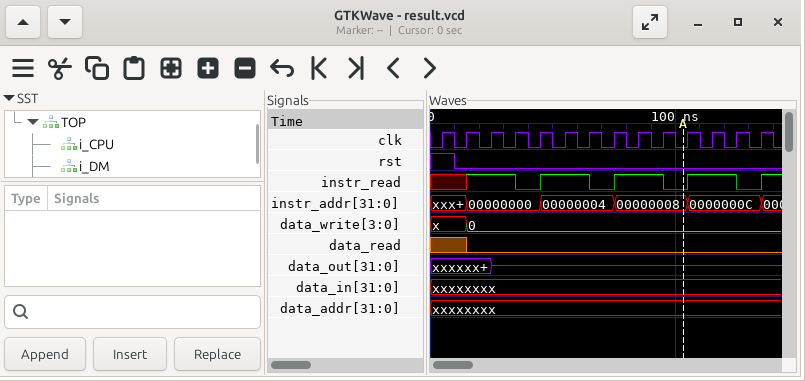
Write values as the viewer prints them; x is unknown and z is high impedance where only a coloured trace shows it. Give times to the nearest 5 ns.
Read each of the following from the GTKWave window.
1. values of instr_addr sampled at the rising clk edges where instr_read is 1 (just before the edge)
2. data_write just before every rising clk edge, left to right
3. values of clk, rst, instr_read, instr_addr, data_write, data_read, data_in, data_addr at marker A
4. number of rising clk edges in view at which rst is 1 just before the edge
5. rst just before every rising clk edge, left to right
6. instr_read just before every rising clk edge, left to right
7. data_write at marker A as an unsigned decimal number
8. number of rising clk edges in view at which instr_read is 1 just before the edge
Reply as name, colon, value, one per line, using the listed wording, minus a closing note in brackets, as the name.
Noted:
values of instr_addr sampled at the rising clk edges where instr_read is 1: 00000000, 00000000, 00000004, 00000004, 00000008, 00000008, 0000000C, 0000000C
data_write just before every rising clk edge, left to right: x, x, 0, 0, 0, 0, 0, 0, 0, 0, 0, 0, 0, 0
values of clk, rst, instr_read, instr_addr, data_write, data_read, data_in, data_addr at marker A: clk=0, rst=0, instr_read=0, instr_addr=00000008, data_write=0, data_read=0, data_in=xxxxxxxx, data_addr=xxxxxxxx
number of rising clk edges in view at which rst is 1 just before the edge: 1
rst just before every rising clk edge, left to right: 1 0 0 0 0 0 0 0 0 0 0 0 0 0
instr_read just before every rising clk edge, left to right: x x 1 1 0 1 1 0 1 1 0 1 1 0
data_write at marker A as an unsigned decimal number: 0
number of rising clk edges in view at which instr_read is 1 just before the edge: 8
